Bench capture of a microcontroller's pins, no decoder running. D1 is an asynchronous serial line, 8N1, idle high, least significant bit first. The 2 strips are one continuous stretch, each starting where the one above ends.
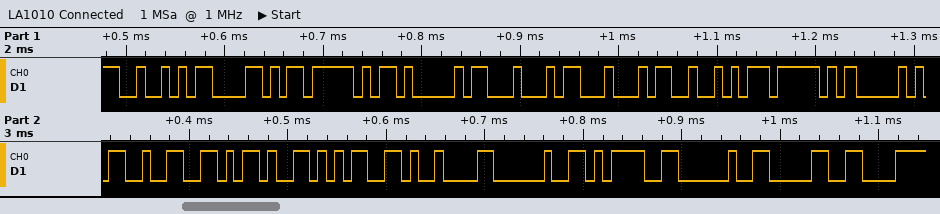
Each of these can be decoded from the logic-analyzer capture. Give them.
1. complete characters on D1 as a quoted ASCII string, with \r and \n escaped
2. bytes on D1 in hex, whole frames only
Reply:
"RX_ADDR_P2-5\t = 0"
0x52 0x58 0x5F 0x41 0x44 0x44 0x52 0x5F 0x50 0x32 0x2D 0x35 0x09 0x20 0x3D 0x20 0x30
